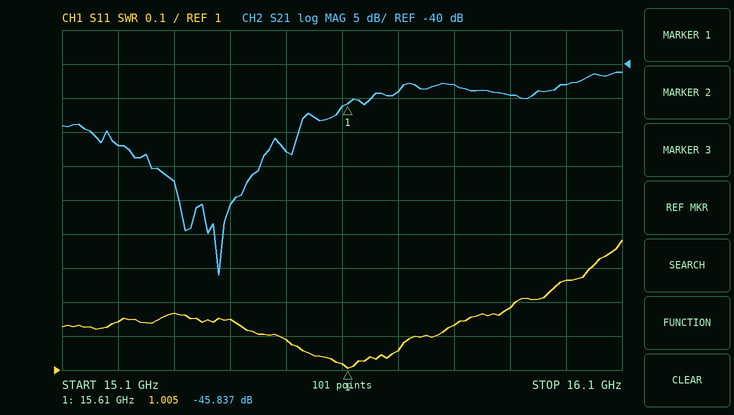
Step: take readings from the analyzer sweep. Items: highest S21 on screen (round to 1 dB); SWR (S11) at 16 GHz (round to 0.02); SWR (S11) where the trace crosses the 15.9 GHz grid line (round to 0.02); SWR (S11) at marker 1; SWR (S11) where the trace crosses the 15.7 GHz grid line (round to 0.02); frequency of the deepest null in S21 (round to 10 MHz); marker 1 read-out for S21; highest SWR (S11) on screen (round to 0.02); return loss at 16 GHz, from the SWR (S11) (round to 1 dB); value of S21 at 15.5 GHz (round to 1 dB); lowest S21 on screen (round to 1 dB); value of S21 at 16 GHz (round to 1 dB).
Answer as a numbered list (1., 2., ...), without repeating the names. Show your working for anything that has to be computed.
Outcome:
1. -41 dB
2. 1.26
3. 1.18
4. 1.005
5. 1.06
6. 15.38 GHz
7. -45.837 dB
8. 1.38
9. −20 log10((1.26 − 1)/(1.26 + 1)) ≈ 19 dB
10. -53 dB
11. -71 dB
12. -43 dB
